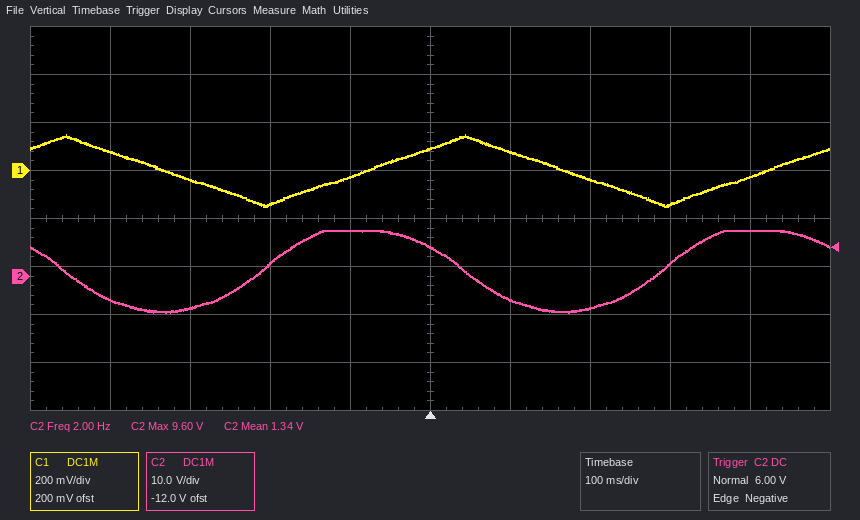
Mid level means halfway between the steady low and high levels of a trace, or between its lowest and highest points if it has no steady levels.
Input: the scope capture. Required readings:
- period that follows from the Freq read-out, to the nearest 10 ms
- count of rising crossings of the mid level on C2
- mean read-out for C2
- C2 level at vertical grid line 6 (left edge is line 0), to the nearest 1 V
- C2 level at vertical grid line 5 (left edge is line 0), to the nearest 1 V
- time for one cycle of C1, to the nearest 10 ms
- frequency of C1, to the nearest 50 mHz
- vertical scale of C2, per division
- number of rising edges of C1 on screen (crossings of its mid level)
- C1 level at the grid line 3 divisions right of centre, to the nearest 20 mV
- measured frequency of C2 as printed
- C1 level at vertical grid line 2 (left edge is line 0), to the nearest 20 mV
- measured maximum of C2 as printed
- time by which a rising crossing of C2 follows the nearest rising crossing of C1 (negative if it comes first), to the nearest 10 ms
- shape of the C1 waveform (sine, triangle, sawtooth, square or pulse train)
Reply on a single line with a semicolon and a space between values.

500 ms; 2; 1.34 V; -5 V; 6 V; 500 ms; 2.00 Hz; 10 V; 2; -140 mV; 2.00 Hz; -40 mV; 9.60 V; -130 ms; triangle
